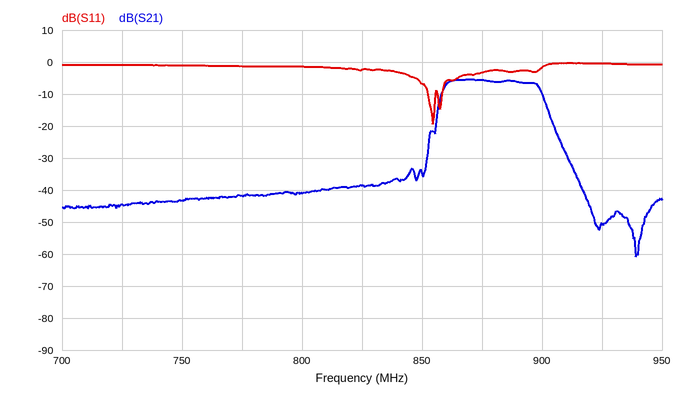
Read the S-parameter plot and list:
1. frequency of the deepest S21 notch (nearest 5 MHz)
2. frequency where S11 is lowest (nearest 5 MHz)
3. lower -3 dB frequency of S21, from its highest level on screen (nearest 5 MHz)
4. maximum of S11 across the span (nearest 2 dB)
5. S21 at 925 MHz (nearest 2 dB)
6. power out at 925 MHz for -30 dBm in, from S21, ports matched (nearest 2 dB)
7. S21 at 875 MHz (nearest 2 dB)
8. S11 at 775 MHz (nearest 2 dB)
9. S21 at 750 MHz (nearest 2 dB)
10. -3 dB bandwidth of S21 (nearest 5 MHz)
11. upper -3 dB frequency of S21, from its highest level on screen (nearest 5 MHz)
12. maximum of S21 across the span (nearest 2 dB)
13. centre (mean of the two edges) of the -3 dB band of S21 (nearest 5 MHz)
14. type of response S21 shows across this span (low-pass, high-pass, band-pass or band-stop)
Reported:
940 MHz
855 MHz
860 MHz
0 dB
-50 dB
-80 dBm
-6 dB
-2 dB
-44 dB
40 MHz
900 MHz
-6 dB
880 MHz
band-pass
